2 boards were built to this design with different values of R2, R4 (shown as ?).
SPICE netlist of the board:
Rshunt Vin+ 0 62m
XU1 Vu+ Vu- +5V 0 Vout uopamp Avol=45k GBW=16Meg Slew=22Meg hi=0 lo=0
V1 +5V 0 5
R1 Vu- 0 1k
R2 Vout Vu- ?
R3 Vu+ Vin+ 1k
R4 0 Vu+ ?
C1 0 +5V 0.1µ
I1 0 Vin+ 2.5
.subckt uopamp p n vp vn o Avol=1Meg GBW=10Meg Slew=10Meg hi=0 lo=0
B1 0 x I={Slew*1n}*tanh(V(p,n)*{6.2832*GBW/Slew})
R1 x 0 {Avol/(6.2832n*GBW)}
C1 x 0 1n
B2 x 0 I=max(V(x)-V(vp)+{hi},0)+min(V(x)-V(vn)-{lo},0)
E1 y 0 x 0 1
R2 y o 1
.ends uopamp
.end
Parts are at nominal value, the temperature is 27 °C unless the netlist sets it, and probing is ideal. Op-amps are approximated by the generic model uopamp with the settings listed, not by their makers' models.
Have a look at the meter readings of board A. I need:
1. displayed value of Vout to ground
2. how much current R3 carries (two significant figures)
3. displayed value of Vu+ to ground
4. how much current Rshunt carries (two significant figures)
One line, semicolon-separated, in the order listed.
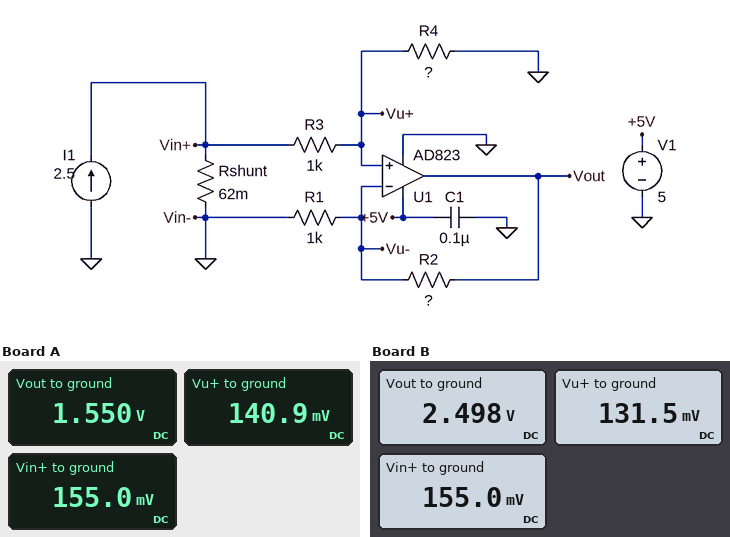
1.550 V; 14 µA; 140.9 mV; 2.5 A
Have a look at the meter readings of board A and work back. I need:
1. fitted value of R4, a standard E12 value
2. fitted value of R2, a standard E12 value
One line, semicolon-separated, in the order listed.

10 kΩ; 10 kΩ
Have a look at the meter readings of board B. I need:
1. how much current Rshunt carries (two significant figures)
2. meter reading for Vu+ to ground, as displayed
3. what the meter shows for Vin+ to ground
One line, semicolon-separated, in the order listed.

2.5 A; 131.5 mV; 155.0 mV
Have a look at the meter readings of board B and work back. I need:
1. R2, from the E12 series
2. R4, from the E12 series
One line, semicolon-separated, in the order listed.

18 kΩ; 5.6 kΩ
